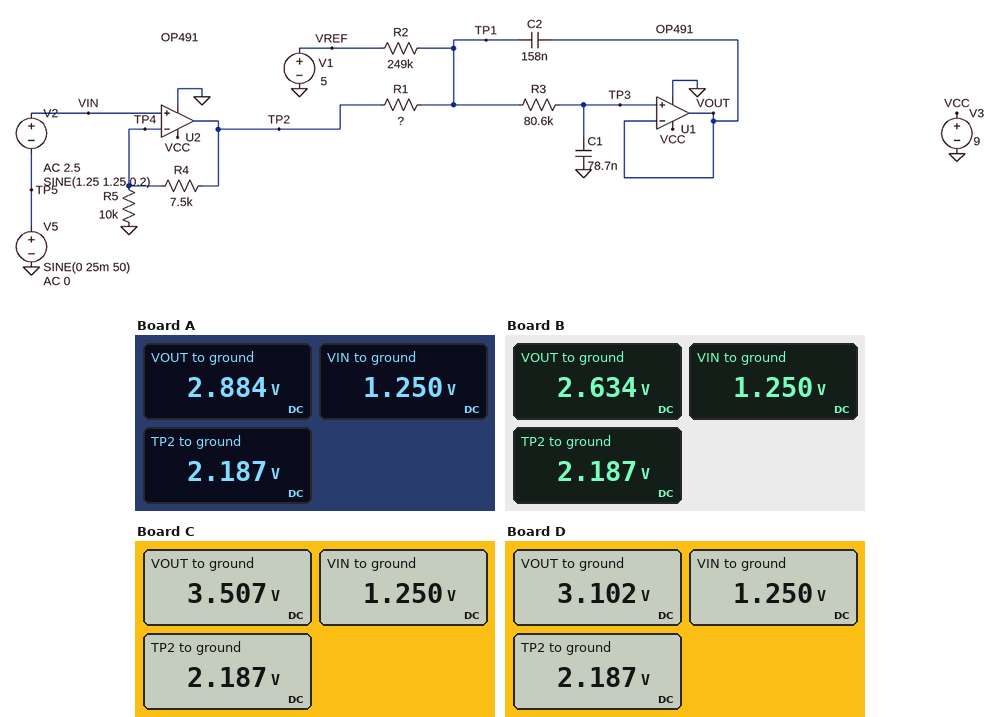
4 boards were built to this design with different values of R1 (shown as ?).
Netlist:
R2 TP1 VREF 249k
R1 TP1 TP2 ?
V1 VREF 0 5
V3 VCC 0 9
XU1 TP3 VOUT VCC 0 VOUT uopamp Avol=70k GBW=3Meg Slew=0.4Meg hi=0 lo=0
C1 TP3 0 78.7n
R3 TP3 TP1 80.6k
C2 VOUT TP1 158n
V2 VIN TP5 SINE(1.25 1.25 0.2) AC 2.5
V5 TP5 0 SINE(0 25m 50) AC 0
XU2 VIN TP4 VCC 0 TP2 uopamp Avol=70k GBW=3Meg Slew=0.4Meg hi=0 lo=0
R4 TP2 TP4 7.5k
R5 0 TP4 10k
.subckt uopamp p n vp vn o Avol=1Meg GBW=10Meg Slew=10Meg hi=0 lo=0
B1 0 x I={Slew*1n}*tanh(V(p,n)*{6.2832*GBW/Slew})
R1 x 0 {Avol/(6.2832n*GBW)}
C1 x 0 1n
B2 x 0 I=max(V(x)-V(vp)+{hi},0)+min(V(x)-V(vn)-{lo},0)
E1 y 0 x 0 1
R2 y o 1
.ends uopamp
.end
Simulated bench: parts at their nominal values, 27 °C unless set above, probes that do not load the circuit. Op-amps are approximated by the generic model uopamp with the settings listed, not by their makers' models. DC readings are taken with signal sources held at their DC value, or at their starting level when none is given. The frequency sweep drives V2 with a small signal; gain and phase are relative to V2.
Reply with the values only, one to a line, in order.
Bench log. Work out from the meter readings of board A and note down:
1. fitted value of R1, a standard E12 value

82 kΩ
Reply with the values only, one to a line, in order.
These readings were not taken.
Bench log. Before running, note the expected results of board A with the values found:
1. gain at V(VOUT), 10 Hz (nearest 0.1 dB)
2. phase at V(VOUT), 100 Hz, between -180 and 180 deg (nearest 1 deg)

2.1 dB
-163 deg
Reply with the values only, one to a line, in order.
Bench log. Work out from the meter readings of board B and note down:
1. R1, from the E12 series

47 kΩ
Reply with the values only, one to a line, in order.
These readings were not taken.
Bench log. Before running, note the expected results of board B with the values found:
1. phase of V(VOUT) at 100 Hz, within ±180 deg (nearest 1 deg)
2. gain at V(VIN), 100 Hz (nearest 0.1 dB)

-158 deg
0 dB
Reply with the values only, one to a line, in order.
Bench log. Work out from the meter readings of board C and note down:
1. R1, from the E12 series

220 kΩ
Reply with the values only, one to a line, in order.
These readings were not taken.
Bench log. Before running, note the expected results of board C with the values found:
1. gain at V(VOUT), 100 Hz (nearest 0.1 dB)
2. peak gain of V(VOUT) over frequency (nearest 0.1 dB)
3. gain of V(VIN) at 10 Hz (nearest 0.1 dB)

-33.9 dB
-0.6 dB
0 dB
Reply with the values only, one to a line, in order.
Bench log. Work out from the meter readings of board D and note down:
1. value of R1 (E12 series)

120 kΩ
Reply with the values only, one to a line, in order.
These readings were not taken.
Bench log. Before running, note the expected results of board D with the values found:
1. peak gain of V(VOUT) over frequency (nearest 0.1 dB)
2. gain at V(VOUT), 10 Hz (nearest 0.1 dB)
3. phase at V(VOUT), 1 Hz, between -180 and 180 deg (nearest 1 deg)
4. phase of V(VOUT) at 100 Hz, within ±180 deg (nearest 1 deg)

1.4 dB
1.0 dB
-5 deg
-166 deg
